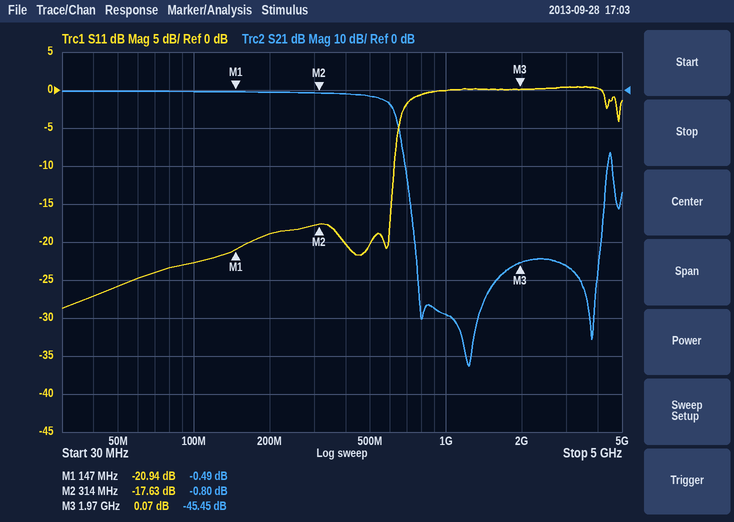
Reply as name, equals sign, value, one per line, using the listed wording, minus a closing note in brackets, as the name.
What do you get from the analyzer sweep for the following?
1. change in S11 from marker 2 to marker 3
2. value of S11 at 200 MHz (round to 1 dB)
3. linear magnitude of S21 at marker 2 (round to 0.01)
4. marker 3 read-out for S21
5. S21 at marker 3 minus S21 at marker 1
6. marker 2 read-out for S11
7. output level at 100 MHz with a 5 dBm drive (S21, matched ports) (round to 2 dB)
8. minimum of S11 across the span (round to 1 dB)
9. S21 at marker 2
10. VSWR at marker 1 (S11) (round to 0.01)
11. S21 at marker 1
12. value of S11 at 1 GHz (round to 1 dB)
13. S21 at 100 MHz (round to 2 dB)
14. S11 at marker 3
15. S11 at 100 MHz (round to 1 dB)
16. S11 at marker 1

change in S11 from marker 2 to marker 3 = 17.70 dB
value of S11 at 200 MHz = -19 dB
linear magnitude of S21 at marker 2 = 0.91
marker 3 read-out for S21 = -45.45 dB
S21 at marker 3 minus S21 at marker 1 = -44.96 dB
marker 2 read-out for S11 = -17.63 dB
output level at 100 MHz with a 5 dBm drive (S21, matched ports) = 4 dBm
minimum of S11 across the span = -29 dB
S21 at marker 2 = -0.80 dB
VSWR at marker 1 (S11) = 1.20
S21 at marker 1 = -0.49 dB
value of S11 at 1 GHz = 0 dB
S21 at 100 MHz = 0 dB
S11 at marker 3 = 0.07 dB
S11 at 100 MHz = -23 dB
S11 at marker 1 = -20.94 dB
